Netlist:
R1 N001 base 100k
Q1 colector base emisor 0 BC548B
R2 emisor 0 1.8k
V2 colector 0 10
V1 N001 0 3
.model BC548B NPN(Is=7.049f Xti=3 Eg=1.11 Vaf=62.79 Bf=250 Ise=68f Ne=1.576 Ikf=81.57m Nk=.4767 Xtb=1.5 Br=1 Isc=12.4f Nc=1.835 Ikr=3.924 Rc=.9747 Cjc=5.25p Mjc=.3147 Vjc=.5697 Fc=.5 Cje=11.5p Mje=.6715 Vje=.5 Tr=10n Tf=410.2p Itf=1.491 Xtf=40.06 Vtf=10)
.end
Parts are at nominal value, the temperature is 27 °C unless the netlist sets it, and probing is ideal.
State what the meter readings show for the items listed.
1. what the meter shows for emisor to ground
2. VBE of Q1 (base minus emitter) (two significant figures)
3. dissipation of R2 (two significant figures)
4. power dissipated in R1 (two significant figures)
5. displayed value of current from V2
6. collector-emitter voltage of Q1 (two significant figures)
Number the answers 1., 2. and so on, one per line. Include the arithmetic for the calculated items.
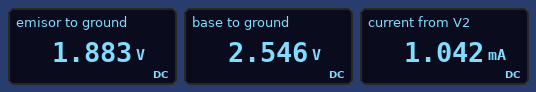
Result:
1. 1.883 V
2. 2.546 V - 1.883 V = 660 mV
3. (1.883 V)^2 / 1.8 kΩ = 2.0 mW
4. (3 V - 2.546 V)^2 / 100 kΩ = 2.1 µW
5. 1.042 mA
6. 10 V - 1.883 V = 8.1 V
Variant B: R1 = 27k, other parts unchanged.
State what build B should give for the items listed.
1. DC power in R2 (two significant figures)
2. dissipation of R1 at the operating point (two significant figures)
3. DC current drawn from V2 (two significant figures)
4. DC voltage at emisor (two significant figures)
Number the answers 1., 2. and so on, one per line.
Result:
1. 2.7 mW
2. 750 nW
3. 1.2 mA
4. 2.2 V
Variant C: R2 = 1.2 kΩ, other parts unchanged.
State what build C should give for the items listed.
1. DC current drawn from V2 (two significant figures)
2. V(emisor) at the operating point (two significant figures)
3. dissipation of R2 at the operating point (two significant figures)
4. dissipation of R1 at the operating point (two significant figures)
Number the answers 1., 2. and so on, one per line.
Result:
1. 1.4 mA
2. 1.7 V
3. 2.5 mW
4. 3.7 µW
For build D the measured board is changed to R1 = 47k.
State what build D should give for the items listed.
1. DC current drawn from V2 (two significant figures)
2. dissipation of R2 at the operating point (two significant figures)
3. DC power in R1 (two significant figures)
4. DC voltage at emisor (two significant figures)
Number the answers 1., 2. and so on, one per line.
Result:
1. 1.2 mA
2. 2.4 mW
3. 1.2 µW
4. 2.1 V
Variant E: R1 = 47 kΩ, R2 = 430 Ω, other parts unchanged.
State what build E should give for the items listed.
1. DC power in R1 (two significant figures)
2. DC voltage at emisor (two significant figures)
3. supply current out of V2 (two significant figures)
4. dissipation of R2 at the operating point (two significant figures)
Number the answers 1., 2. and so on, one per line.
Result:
1. 11 µW
2. 1.6 V
3. 3.7 mA
4. 5.8 mW
